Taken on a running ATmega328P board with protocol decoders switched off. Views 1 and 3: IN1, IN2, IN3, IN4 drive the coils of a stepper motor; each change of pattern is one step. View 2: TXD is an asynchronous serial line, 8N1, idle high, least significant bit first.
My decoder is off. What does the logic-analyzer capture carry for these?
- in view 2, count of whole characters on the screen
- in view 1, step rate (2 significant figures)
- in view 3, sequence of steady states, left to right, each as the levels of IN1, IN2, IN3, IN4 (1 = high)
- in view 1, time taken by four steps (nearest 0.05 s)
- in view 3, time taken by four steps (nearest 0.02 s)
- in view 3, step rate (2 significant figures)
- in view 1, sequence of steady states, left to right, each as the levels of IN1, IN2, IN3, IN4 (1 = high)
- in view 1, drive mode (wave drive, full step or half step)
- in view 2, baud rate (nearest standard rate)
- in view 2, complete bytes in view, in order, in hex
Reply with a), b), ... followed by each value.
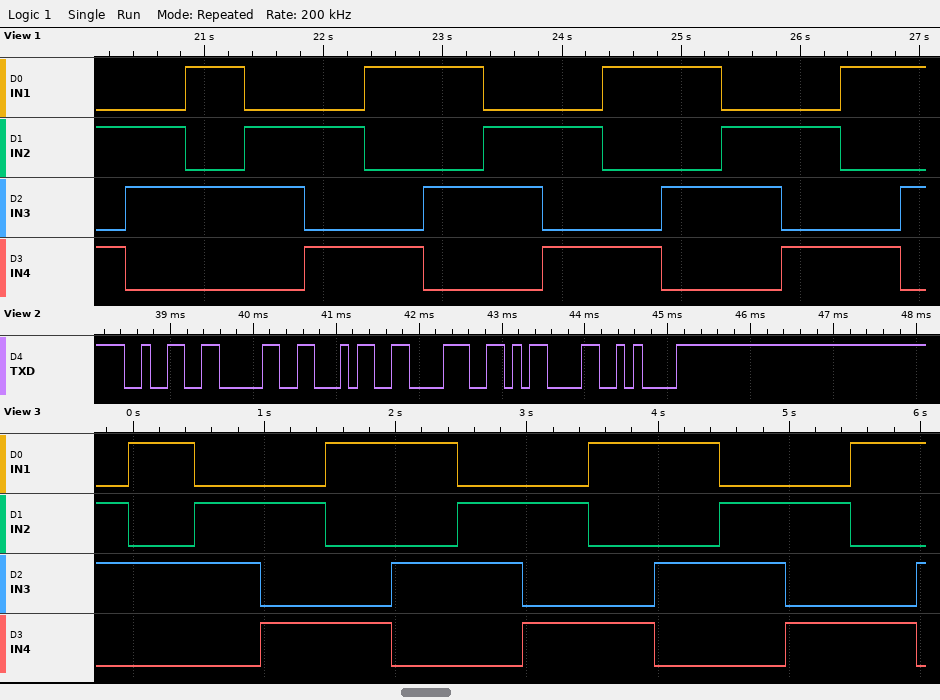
a) 6
b) 2.0 steps/s
c) 0110 1010 0110 0101 1001 1010 0110 0101 1001 1010 0110 0101 1001 1010
d) 2.00 s
e) 2.00 s
f) 2.0 steps/s
g) 0101 0110 1010 0110 0101 1001 1010 0110 0101 1001 1010 0110 0101 1001 1010
h) full step
i) 9600 baud
j) 32 30 34 38 0D 0A
